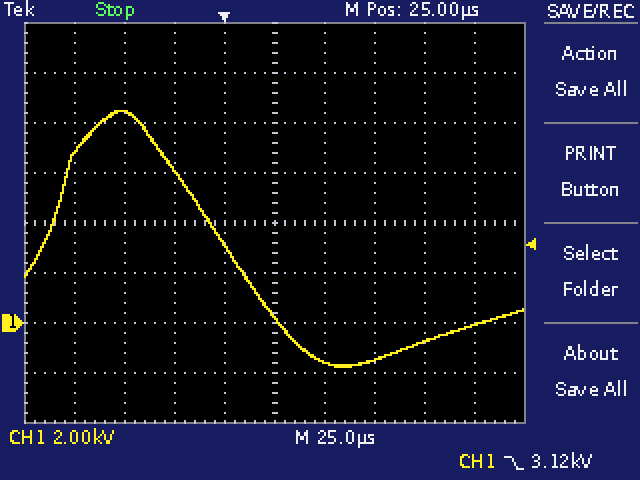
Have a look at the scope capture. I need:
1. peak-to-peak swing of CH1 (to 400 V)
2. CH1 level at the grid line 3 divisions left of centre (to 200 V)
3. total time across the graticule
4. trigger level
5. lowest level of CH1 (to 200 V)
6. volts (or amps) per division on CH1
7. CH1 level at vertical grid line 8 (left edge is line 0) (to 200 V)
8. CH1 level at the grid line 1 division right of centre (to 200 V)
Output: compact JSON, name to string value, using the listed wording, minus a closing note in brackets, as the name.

{"peak-to-peak swing of CH1": "10.4 kV", "CH1 level at the grid line 3 divisions left of centre": "8.4 kV", "total time across the graticule": "250 µs", "trigger level": "3.12 kV", "lowest level of CH1": "-1.8 kV", "volts (or amps) per division on CH1": "2 kV", "CH1 level at vertical grid line 8 (left edge is line 0)": "-800 V", "CH1 level at the grid line 1 division right of centre": "-1.6 kV"}
